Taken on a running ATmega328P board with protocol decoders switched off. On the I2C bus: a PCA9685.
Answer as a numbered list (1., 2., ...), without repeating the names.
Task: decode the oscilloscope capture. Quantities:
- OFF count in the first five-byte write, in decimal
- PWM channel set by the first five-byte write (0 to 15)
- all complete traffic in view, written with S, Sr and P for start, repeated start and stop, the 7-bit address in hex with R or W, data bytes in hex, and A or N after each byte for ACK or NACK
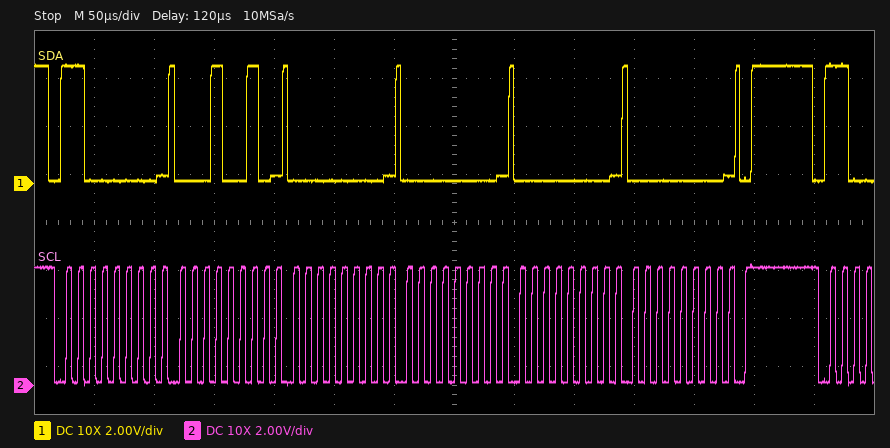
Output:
1. 0
2. 3
3. S 60W A 12 A 00 A 00 A 00 A 00 A P
